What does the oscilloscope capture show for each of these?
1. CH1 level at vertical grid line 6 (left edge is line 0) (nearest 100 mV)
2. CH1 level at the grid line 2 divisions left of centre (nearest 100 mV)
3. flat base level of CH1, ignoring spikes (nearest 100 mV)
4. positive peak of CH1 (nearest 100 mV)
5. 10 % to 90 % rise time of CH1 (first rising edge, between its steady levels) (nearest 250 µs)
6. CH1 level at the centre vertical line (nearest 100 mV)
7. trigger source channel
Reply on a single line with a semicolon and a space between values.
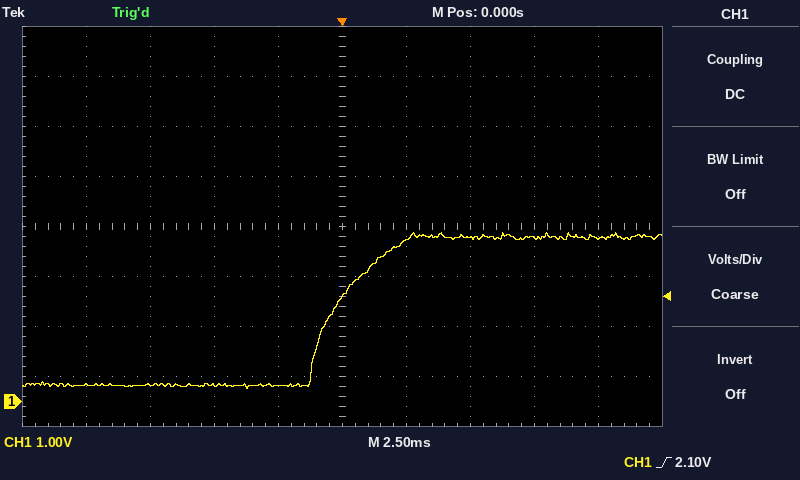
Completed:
3.2 V; 300 mV; 300 mV; 3.4 V; 3.00 ms; 2.1 V; CH1
